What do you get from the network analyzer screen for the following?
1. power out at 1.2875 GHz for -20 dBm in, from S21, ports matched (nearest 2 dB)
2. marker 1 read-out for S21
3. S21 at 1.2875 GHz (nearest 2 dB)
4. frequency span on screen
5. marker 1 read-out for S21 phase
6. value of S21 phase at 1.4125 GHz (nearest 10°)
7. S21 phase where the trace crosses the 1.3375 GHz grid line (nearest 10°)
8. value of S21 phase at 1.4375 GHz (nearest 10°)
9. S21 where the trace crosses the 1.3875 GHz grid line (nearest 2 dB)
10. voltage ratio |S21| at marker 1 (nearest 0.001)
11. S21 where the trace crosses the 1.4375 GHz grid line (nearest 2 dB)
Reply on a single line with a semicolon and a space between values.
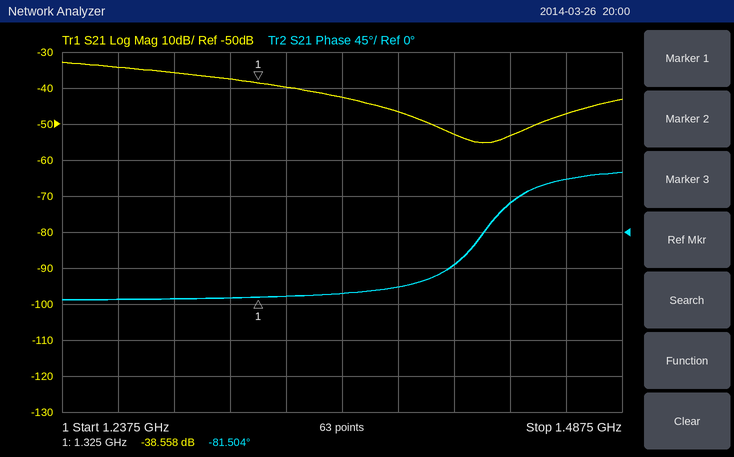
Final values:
-56 dBm; -38.558 dB; -36 dB; 250 MHz; -81.504°; -40°; -80°; 40°; -46 dB; 0.012; -54 dB
